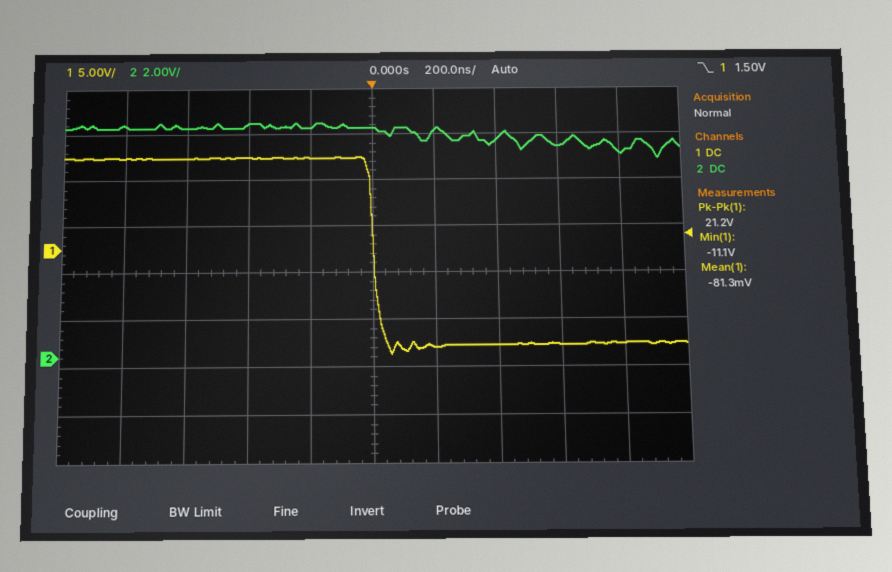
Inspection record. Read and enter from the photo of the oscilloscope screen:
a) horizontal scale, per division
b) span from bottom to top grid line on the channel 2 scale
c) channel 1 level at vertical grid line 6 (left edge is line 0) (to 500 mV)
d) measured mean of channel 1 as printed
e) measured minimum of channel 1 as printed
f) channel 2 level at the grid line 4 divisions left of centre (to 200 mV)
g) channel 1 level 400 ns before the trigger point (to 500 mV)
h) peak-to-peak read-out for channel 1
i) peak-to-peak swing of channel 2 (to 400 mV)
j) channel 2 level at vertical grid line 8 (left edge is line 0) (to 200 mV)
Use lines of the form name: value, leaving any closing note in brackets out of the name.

horizontal scale, per division: 200 ns
span from bottom to top grid line on the channel 2 scale: 16 V
channel 1 level at vertical grid line 6 (left edge is line 0): -10.5 V
measured mean of channel 1 as printed: -81.3 mV
measured minimum of channel 1 as printed: -11.1 V
channel 2 level at the grid line 4 divisions left of centre: 10.0 V
channel 1 level 400 ns before the trigger point: 10.0 V
peak-to-peak read-out for channel 1: 21.2 V
peak-to-peak swing of channel 2: 1.6 V
channel 2 level at vertical grid line 8 (left edge is line 0): 9.0 V
